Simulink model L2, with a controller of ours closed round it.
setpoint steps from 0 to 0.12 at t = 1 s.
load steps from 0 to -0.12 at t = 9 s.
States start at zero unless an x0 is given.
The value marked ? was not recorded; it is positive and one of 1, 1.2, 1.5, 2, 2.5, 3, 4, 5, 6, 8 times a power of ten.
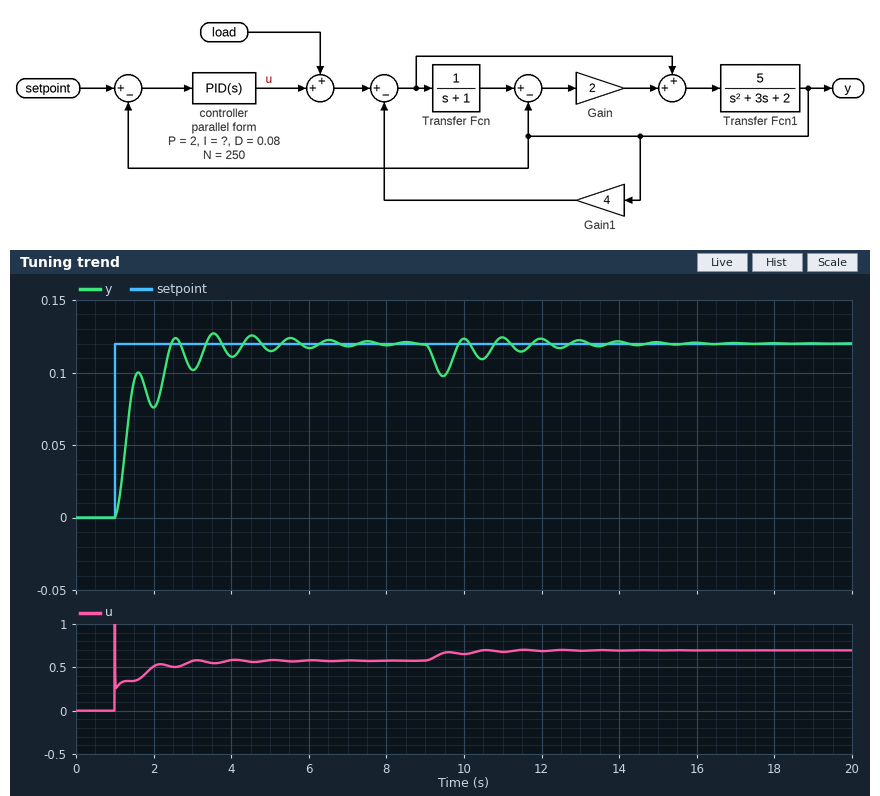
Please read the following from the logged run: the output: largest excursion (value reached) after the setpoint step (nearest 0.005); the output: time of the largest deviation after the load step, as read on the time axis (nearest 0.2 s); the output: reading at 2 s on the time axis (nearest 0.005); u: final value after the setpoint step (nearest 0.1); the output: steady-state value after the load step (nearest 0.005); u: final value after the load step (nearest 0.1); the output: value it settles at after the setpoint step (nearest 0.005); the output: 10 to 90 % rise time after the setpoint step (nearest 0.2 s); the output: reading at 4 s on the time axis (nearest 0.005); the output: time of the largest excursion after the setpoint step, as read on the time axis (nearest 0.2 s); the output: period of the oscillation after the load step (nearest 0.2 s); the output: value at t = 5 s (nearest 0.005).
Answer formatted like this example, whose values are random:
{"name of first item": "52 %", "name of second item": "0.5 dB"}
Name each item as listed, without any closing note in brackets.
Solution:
{"the output: largest excursion (value reached) after the setpoint step": "0.125", "the output: time of the largest deviation after the load step, as read on the time axis": "9.4 s", "the output: reading at 2 s on the time axis": "0.075", "u: final value after the setpoint step": "0.6", "the output: steady-state value after the load step": "0.120", "u: final value after the load step": "0.7", "the output: value it settles at after the setpoint step": "0.120", "the output: 10 to 90 % rise time after the setpoint step": "1.2 s", "the output: reading at 4 s on the time axis": "0.110", "the output: time of the largest excursion after the setpoint step, as read on the time axis": "3.6 s", "the output: period of the oscillation after the load step": "1.0 s", "the output: value at t = 5 s": "0.115"}
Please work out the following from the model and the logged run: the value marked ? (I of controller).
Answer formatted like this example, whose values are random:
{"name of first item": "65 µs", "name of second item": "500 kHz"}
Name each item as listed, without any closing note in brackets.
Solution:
{"the value marked ?": "8"}
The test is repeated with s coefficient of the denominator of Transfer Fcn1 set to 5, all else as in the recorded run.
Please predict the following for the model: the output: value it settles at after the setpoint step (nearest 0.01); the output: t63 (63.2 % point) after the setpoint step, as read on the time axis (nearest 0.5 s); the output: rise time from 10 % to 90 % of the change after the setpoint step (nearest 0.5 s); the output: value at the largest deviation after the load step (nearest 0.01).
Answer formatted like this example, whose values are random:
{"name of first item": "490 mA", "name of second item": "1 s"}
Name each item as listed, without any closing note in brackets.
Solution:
{"the output: value it settles at after the setpoint step": "0.12", "the output: t63 (63.2 % point) after the setpoint step, as read on the time axis": "1.5 s", "the output: rise time from 10 % to 90 % of the change after the setpoint step": "1.5 s", "the output: value at the largest deviation after the load step": "0.10"}
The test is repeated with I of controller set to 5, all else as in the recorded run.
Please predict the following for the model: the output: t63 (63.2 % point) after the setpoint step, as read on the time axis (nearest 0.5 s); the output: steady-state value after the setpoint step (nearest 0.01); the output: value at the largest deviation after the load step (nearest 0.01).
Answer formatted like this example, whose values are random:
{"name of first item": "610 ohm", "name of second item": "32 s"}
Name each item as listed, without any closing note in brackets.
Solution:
{"the output: t63 (63.2 % point) after the setpoint step, as read on the time axis": "1.5 s", "the output: steady-state value after the setpoint step": "0.12", "the output: value at the largest deviation after the load step": "0.10"}
